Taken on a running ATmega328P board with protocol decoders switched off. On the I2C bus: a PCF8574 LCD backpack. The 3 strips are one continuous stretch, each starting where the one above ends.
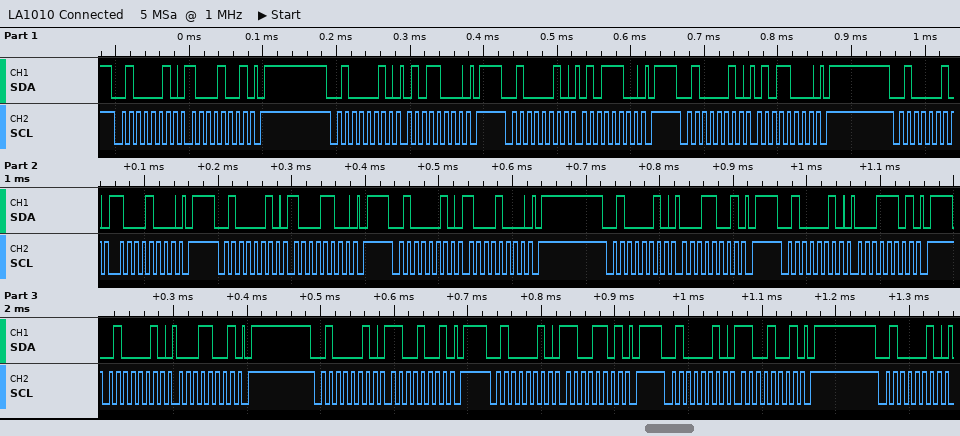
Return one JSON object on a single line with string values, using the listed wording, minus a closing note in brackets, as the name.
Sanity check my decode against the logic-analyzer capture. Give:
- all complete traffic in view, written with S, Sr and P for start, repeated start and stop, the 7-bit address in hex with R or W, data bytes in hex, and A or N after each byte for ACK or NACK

{"all complete traffic in view, written with S, Sr and P for start, repeated start and stop, the 7-bit address in hex with R or W, data bytes in hex, and A or N after each byte for ACK or NACK": "S 21W A 89 A P S 21W A 58 A P S 21W A 5C A P S 21W A 58 A P S 21W A 88 A P S 21W A 8C A P S 21W A 88 A P S 21W A 19 A P S 21W A 1D A P S 21W A 19 A P S 21W A C9 A P S 21W A CD A P S 21W A C9 A P S 21W A"}
